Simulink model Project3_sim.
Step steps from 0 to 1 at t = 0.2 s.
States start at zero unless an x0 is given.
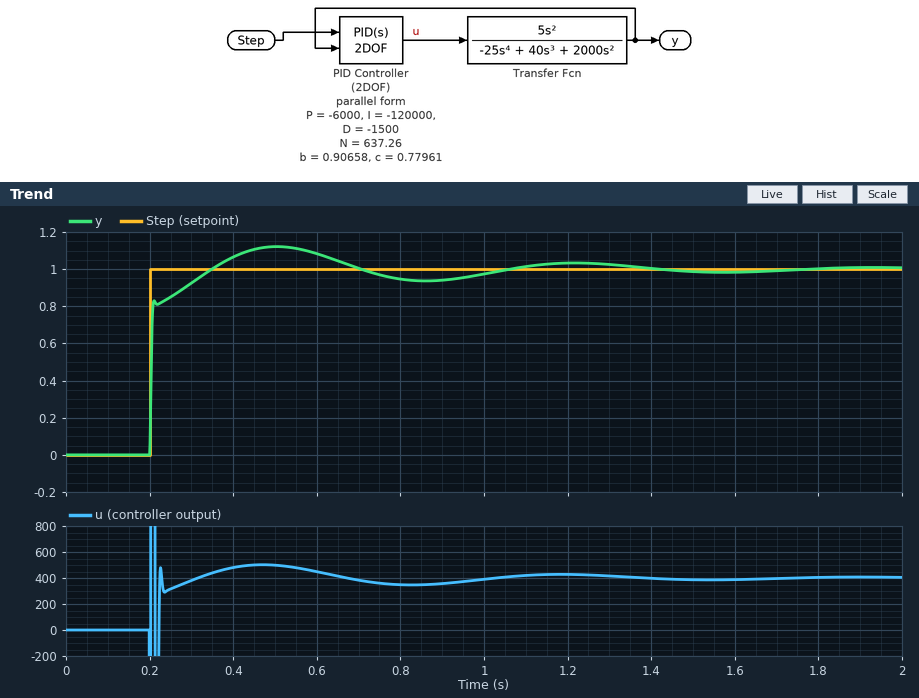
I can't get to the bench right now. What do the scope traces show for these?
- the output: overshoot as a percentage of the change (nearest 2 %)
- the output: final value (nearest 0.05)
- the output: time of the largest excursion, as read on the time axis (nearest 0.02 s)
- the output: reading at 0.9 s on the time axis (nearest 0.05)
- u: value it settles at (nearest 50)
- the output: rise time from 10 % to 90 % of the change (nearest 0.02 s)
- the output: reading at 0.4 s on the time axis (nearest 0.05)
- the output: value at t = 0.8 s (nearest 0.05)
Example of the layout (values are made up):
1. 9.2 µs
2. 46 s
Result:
1. 12 %
2. 1.00
3. 0.50 s
4. 0.95
5. 400
6. 0.08 s
7. 1.05
8. 0.95
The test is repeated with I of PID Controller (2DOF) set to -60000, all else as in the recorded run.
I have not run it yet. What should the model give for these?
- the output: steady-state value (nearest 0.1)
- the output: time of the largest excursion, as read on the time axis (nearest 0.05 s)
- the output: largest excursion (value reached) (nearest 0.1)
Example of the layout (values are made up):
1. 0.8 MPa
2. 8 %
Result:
1. 1.0
2. 0.60 s
3. 1.1
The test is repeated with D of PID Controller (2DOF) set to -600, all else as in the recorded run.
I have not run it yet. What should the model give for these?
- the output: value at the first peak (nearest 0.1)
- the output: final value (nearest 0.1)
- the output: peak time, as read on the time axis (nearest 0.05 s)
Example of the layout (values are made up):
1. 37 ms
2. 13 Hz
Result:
1. 1.1
2. 1.0
3. 0.35 s
